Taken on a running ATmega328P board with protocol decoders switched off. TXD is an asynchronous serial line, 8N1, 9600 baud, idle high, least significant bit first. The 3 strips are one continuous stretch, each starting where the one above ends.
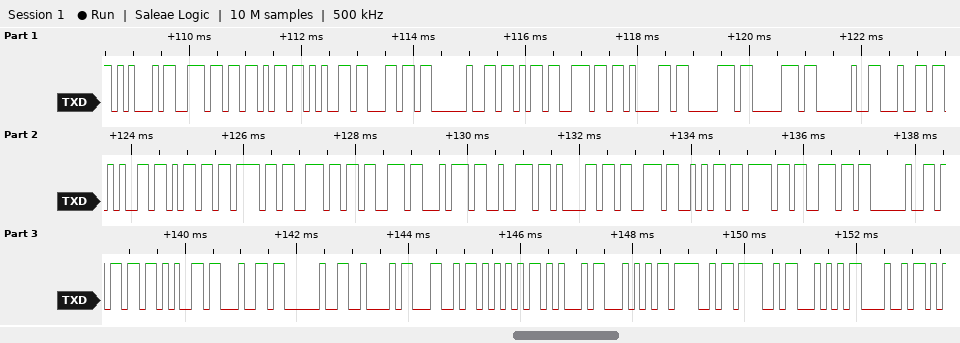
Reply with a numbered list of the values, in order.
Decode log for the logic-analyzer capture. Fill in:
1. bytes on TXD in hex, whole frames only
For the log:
1. 45 6E 6B 65 6C 20 6B 6E 61 70 70 20 64 65 6D 6F 6E 73 74 72 61 73 6A 6F 6E 20 6D 65 64 20 42 4C 55 45 54 4F 4F 54 48
